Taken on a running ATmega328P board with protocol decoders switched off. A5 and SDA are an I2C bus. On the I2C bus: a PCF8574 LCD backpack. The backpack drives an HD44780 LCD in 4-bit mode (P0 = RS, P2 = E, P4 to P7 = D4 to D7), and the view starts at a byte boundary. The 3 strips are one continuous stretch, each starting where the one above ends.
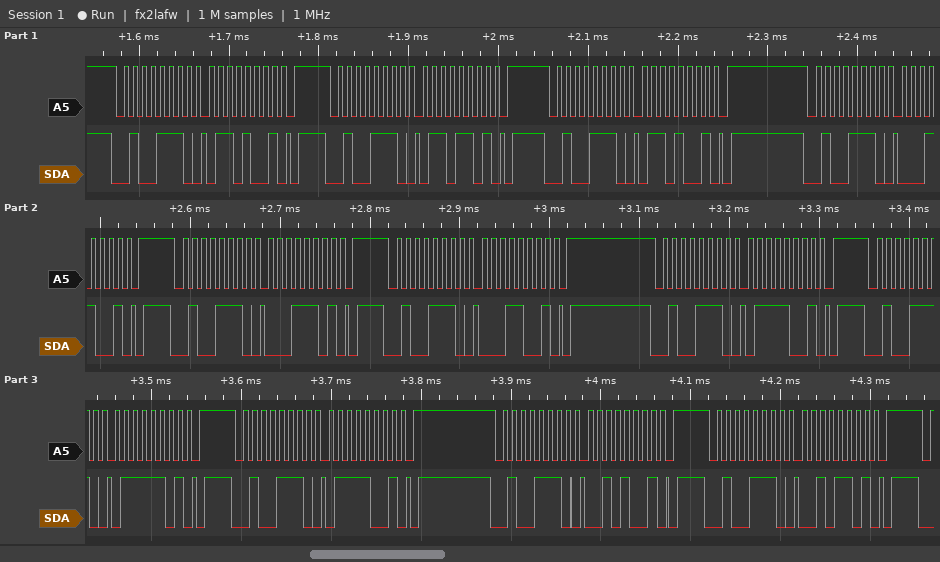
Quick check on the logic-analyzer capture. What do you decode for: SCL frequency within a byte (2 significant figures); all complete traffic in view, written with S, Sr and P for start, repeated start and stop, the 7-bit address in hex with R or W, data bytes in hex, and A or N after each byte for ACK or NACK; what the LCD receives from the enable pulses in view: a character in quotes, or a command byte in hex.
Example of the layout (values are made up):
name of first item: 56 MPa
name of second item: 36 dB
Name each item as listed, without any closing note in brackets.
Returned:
SCL frequency within a byte: 100 kHz
all complete traffic in view, written with S, Sr and P for start, repeated start and stop, the 7-bit address in hex with R or W, data bytes in hex, and A or N after each byte for ACK or NACK: S 27W A 69 A P S 27W A 6D A P S 27W A 69 A P S 27W A 19 A P S 27W A 1D A P S 27W A 19 A P S 27W A 79 A P S 27W A 7D A P S 27W A 79 A P S 27W A 29 A P S 27W A 2D A P
what the LCD receives from the enable pulses in view: a character in quotes, or a command byte in hex: 'a'
